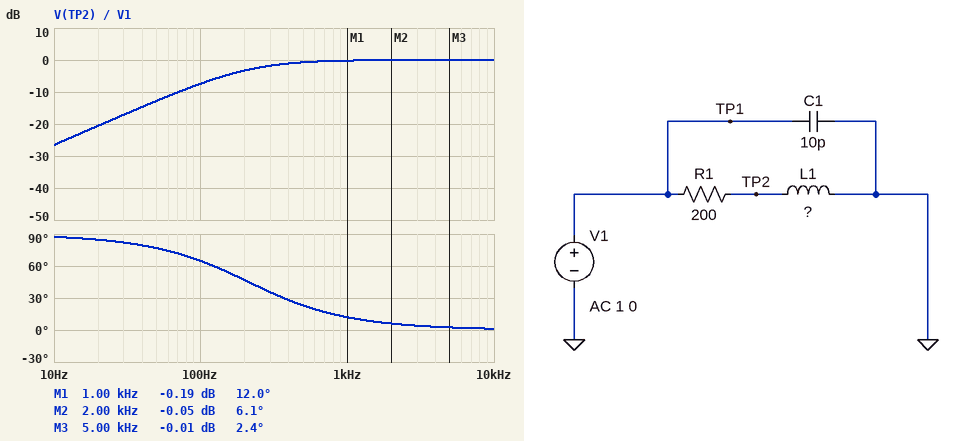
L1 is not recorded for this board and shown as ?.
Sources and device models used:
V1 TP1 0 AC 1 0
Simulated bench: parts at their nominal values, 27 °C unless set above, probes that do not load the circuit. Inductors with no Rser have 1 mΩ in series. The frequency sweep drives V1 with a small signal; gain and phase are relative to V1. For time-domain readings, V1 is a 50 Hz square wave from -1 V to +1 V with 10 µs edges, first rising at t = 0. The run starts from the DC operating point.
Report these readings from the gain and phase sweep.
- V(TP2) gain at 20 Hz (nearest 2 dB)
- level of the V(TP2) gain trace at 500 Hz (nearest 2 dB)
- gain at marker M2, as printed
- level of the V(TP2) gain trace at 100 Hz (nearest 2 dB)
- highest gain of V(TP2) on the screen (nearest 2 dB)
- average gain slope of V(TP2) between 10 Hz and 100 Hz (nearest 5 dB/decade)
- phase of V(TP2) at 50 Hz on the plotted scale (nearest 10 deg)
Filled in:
-20 dB
0 dB
-0.05 dB
-8 dB
0 dB
20 dB/decade
80 deg
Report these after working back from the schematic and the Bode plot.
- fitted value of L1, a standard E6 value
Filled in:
150 mH
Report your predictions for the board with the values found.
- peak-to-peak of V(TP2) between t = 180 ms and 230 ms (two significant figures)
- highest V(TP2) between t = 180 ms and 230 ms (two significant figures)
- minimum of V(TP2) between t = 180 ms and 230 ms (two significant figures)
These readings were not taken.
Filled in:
4.0 V
2.0 V
-2.0 V
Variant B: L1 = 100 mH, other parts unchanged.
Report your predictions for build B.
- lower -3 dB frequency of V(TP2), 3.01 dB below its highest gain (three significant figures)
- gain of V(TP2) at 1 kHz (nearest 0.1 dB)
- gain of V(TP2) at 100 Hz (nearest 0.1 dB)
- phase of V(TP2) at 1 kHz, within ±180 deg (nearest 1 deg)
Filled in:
318 Hz
-0.4 dB
-10.5 dB
18 deg
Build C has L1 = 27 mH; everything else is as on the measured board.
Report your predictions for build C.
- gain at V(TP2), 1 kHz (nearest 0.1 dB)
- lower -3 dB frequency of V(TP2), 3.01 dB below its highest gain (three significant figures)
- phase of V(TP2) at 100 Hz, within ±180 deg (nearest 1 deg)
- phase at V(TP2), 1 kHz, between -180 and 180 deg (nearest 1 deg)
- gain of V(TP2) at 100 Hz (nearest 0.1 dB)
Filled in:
-3.8 dB
1.18 kHz
85 deg
50 deg
-21.5 dB
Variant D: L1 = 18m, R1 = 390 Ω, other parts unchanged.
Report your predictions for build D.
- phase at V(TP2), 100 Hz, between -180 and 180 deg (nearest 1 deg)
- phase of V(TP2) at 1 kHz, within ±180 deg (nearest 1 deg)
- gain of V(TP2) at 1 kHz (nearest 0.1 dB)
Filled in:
88 deg
74 deg
-11.1 dB
